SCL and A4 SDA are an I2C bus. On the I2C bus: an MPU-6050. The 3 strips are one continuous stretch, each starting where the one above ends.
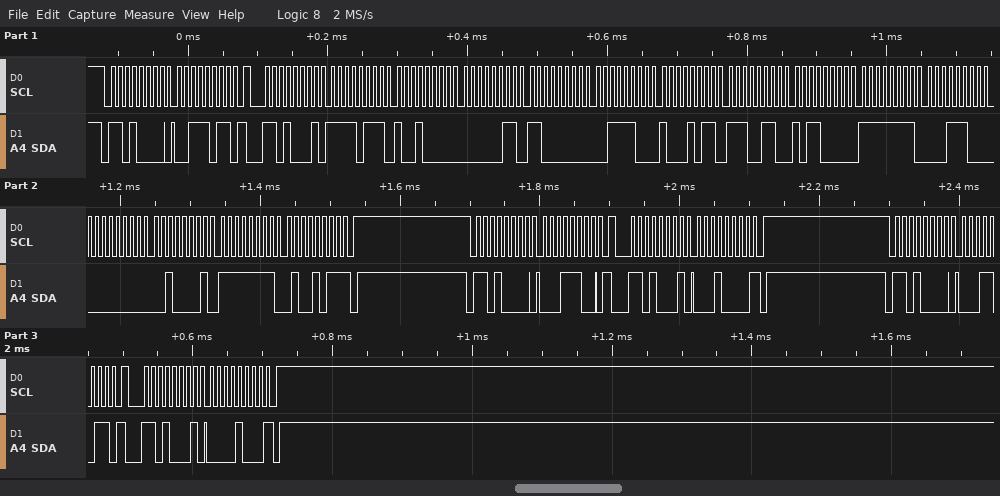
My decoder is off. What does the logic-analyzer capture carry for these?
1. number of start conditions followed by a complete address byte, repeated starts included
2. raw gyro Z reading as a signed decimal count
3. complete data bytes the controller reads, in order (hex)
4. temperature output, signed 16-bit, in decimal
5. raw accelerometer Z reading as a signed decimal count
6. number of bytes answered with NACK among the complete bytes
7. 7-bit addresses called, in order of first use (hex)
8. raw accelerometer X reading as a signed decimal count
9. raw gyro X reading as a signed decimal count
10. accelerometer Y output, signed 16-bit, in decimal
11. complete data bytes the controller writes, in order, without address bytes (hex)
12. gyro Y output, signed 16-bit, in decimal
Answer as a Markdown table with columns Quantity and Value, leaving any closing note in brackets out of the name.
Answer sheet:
| Quantity | Value |
|---|---|
| number of start conditions followed by a complete address byte, repeated starts included | 6 |
| raw gyro Z reading as a signed decimal count | -181 |
| complete data bytes the controller reads, in order | F7 90 03 C0 3C 8B E6 B0 FF 1C 00 21 FF 4B 10 08 |
| temperature output, signed 16-bit, in decimal | -6480 |
| raw accelerometer Z reading as a signed decimal count | 15499 |
| number of bytes answered with NACK among the complete bytes | 3 |
| 7-bit addresses called, in order of first use | 0x68 |
| raw accelerometer X reading as a signed decimal count | -2160 |
| raw gyro X reading as a signed decimal count | -228 |
| accelerometer Y output, signed 16-bit, in decimal | 960 |
| complete data bytes the controller writes, in order, without address bytes | 3B 1C 1B |
| gyro Y output, signed 16-bit, in decimal | 33 |
